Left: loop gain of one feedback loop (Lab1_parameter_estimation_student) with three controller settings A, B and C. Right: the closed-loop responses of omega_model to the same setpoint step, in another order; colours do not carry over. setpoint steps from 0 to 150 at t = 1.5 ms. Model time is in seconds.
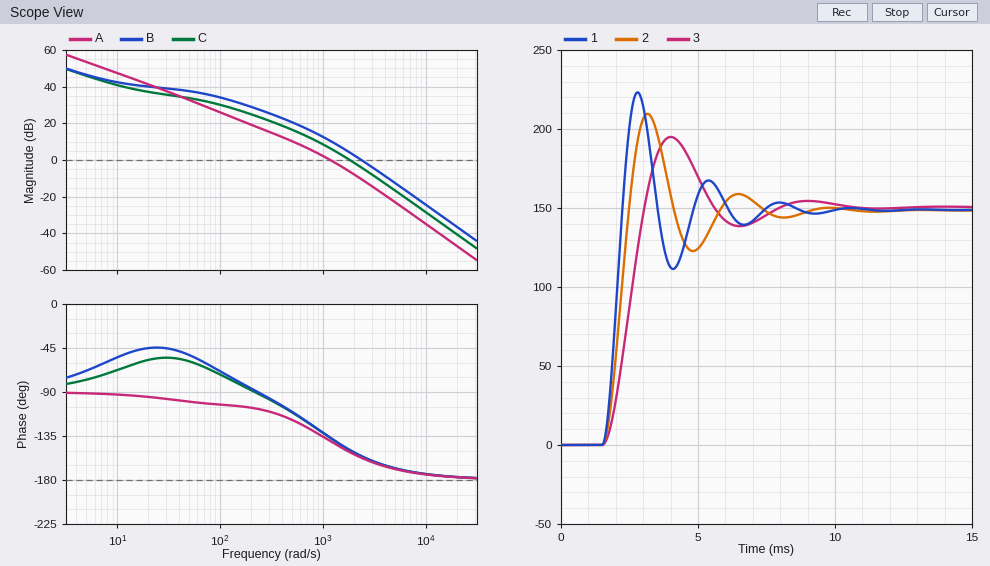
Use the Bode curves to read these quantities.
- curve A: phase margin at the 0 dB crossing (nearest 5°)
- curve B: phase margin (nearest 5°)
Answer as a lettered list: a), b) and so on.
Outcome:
a) 40°
b) 25°
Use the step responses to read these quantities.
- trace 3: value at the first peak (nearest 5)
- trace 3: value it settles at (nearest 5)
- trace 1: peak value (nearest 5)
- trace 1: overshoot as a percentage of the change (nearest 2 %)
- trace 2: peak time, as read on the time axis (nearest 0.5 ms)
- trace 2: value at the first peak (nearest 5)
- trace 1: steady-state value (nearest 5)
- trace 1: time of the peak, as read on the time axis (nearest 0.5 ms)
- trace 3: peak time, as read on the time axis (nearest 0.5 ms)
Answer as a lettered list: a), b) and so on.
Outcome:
a) 195
b) 150
c) 225
d) 50 %
e) 3.0 ms
f) 210
g) 150
h) 3.0 ms
i) 4.0 ms
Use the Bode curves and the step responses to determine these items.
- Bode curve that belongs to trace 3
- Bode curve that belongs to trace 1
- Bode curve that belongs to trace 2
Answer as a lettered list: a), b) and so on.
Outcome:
a) A
b) B
c) C
